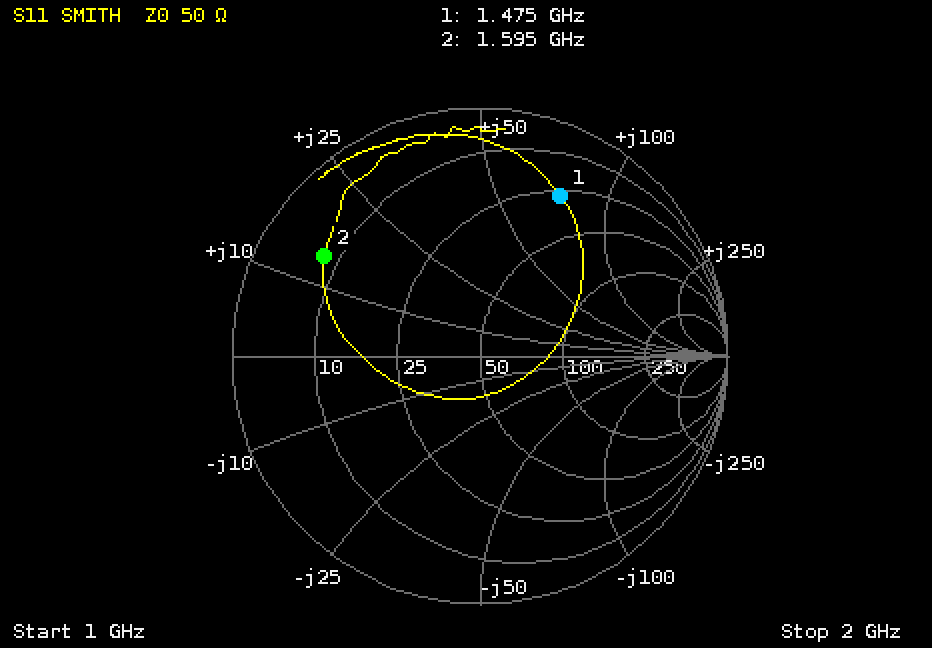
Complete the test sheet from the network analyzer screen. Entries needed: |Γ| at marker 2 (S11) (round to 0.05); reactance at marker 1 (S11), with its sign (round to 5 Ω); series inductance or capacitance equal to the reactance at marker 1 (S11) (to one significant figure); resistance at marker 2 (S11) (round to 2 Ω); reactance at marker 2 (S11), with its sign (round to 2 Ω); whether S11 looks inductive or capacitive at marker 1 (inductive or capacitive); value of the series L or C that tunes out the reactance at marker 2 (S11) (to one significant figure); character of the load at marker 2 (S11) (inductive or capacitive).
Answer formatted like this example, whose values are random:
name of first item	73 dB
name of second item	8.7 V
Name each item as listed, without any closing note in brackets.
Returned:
|Γ| at marker 2 (S11)	0.75
reactance at marker 1 (S11), with its sign	+75 Ω
series inductance or capacitance equal to the reactance at marker 1 (S11)	8 nH
resistance at marker 2 (S11)	8 Ω
reactance at marker 2 (S11), with its sign	+14 Ω
whether S11 looks inductive or capacitive at marker 1	inductive
value of the series L or C that tunes out the reactance at marker 2 (S11)	7 pF
character of the load at marker 2 (S11)	inductive
